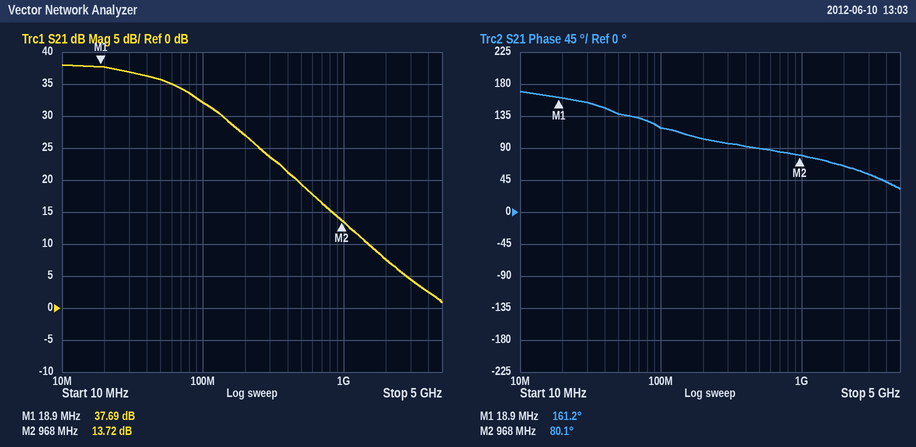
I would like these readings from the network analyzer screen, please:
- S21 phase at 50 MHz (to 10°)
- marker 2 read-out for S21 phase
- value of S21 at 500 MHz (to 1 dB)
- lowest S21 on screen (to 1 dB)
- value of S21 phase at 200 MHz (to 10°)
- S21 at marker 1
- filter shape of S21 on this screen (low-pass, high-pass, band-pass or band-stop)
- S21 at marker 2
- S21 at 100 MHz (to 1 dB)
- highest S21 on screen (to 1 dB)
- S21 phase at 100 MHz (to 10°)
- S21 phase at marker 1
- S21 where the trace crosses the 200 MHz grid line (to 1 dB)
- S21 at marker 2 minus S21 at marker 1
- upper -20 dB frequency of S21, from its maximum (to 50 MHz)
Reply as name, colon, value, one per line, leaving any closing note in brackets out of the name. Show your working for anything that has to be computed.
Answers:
S21 phase at 50 MHz: 140°
marker 2 read-out for S21 phase: 80.1°
value of S21 at 500 MHz: 19 dB
lowest S21 on screen: 1 dB
value of S21 phase at 200 MHz: 100°
S21 at marker 1: 37.69 dB
filter shape of S21 on this screen: low-pass
S21 at marker 2: 13.72 dB
S21 at 100 MHz: 32 dB
highest S21 on screen: 38 dB
S21 phase at 100 MHz: 120°
S21 phase at marker 1: 161.2°
S21 where the trace crosses the 200 MHz grid line: 27 dB
S21 at marker 2 minus S21 at marker 1: 13.72 − (37.69) = -23.97 dB
upper -20 dB frequency of S21, from its maximum: 600 MHz
